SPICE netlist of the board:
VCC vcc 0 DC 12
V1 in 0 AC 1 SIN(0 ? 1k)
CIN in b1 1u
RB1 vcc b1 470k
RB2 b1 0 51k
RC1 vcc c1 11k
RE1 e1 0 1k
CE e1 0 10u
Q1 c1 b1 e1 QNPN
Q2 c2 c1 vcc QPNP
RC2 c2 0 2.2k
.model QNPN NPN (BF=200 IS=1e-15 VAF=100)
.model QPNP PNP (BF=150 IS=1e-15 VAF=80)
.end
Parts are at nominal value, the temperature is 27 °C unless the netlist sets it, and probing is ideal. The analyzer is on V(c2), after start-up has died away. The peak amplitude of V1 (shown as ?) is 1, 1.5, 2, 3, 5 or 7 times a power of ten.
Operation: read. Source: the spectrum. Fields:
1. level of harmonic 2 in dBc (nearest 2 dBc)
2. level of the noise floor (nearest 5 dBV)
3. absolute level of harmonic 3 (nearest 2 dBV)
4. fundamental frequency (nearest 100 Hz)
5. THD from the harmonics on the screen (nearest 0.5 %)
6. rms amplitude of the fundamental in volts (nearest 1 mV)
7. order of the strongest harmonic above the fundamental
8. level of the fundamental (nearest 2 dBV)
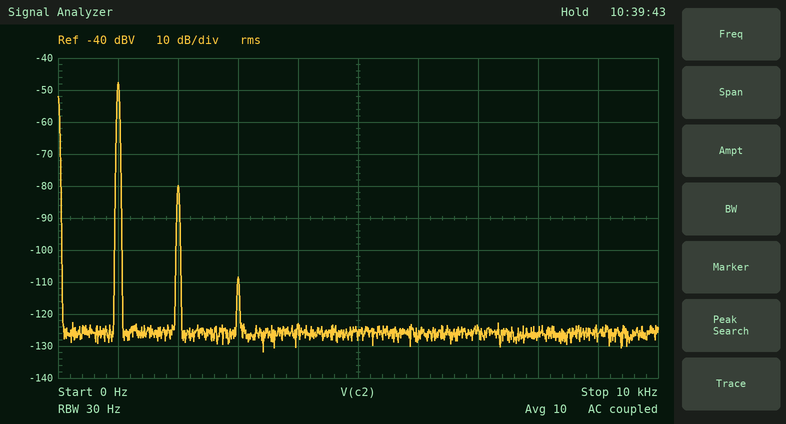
-32 dBc
-125 dBV
-108 dBV
1.0 kHz
2.5 %
4 mV
2
-48 dBV
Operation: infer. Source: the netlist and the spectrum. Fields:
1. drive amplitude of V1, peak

5 mV
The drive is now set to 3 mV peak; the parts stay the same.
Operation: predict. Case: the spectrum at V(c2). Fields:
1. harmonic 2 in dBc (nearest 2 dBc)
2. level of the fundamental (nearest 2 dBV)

-36 dBc
-52 dBV
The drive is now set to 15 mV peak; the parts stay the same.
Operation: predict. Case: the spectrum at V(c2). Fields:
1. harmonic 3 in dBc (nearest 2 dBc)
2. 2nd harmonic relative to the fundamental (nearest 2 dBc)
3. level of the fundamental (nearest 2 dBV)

-40 dBc
-22 dBc
-38 dBV
